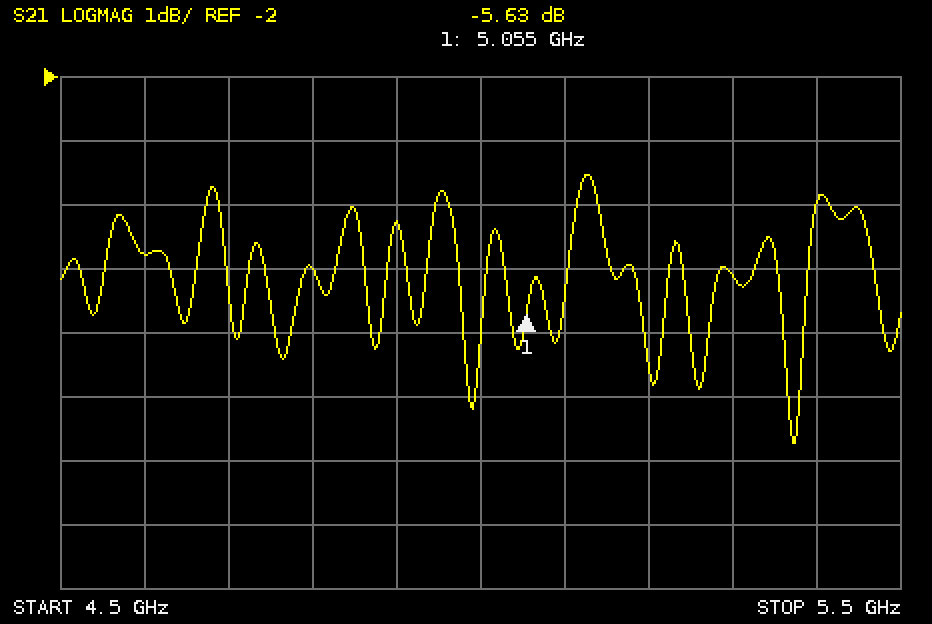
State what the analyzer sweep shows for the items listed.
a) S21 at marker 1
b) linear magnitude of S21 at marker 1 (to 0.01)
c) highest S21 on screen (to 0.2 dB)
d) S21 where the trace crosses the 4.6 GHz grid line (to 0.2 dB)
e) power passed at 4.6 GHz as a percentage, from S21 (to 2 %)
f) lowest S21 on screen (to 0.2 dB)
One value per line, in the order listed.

-5.63 dB
0.52
-3.6 dB
-4.8 dB
34 %
-7.8 dB
